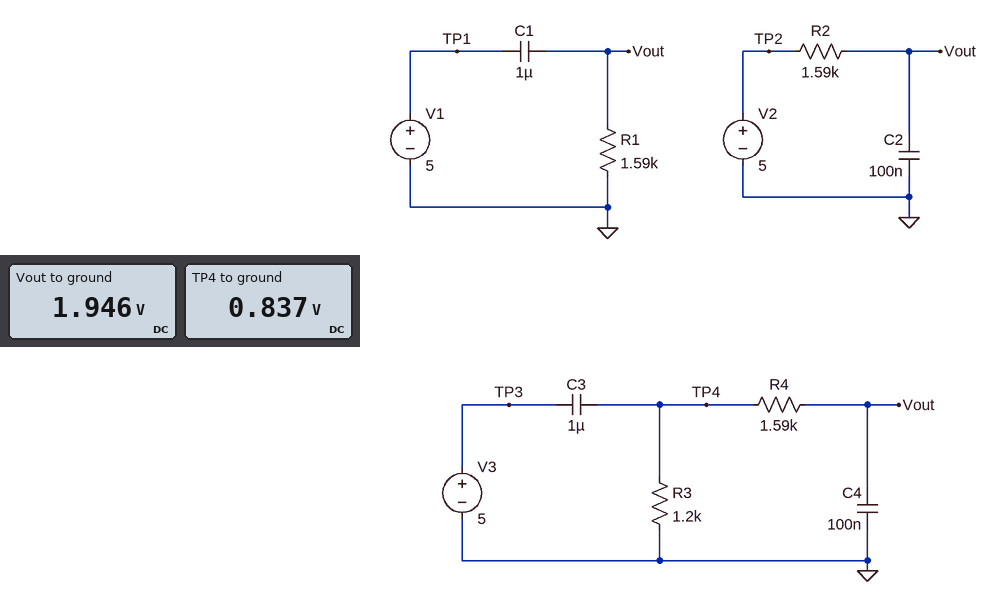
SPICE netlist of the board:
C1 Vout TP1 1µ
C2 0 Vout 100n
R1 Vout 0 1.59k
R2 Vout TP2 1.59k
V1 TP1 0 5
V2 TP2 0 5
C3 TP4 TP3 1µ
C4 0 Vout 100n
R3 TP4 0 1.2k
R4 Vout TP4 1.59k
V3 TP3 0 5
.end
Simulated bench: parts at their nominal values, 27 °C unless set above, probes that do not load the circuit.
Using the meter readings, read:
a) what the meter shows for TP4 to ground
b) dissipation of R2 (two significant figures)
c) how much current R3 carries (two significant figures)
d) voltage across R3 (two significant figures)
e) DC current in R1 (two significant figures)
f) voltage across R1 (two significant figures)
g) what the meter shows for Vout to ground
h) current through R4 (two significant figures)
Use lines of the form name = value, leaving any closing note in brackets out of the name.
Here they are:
what the meter shows for TP4 to ground = 0.837 V
dissipation of R2 = 5.9 mW
how much current R3 carries = 700 µA
voltage across R3 = 840 mV
DC current in R1 = 1.2 mA
voltage across R1 = 1.9 V
what the meter shows for Vout to ground = 1.946 V
current through R4 = 700 µA
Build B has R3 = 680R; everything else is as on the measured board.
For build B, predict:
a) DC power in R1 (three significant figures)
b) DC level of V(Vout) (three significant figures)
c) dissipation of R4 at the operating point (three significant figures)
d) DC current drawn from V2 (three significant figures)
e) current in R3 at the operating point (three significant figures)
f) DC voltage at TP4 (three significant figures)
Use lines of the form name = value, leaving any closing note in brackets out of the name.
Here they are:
DC power in R1 = 2.16 mW
DC level of V(Vout) = 1.85 V
dissipation of R4 at the operating point = 1.06 mW
DC current drawn from V2 = 1.98 mA
current in R3 at the operating point = 816 µA
DC voltage at TP4 = 555 mV
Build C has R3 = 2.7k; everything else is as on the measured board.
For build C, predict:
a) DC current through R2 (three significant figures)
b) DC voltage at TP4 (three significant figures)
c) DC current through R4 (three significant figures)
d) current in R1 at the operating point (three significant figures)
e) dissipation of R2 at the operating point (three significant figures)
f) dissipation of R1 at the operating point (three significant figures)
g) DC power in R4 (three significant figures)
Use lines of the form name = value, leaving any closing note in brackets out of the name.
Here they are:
DC current through R2 = 1.82 mA
DC voltage at TP4 = 1.33 V
DC current through R4 = 492 µA
current in R1 at the operating point = 1.33 mA
dissipation of R2 at the operating point = 5.26 mW
dissipation of R1 at the operating point = 2.80 mW
DC power in R4 = 384 µW
